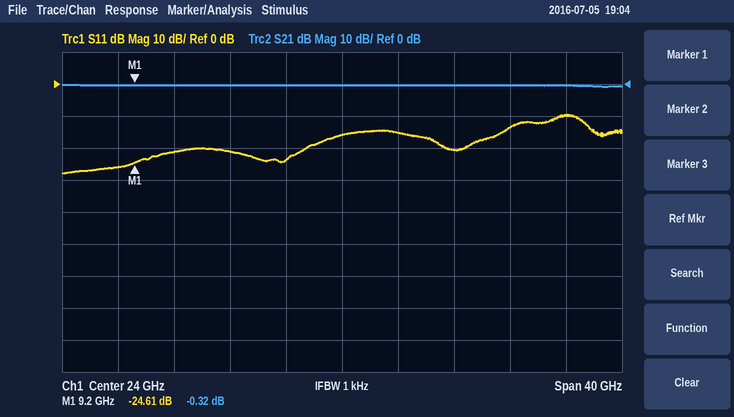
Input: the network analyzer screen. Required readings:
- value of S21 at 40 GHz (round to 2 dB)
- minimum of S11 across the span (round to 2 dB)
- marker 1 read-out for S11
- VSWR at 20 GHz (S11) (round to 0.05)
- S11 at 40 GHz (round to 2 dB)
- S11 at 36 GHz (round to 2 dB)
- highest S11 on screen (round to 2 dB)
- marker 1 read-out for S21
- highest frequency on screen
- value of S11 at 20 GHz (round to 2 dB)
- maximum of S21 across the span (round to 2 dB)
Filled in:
0 dB
-28 dB
-24.61 dB
1.15
-10 dB
-14 dB
-10 dB
-0.32 dB
44 GHz
-24 dB
0 dB
